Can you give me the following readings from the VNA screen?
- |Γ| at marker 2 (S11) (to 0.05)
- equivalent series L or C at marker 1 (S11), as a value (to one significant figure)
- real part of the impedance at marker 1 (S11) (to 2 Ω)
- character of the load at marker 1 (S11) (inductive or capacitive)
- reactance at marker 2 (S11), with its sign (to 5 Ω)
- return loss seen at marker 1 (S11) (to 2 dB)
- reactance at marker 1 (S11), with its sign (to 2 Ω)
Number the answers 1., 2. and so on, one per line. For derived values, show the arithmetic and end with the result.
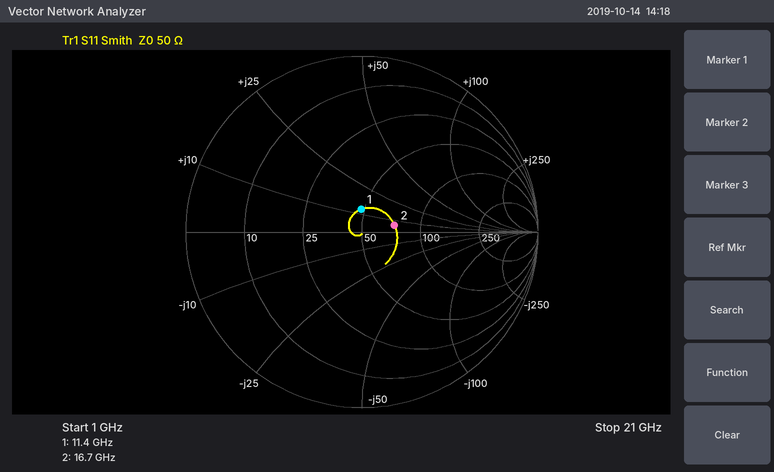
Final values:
1. 0.20
2. L = 12 Ω/(2π × 11.4 GHz) ≈ 168 pH, so 200 pH to one significant figure
3. 48 Ω
4. inductive
5. +5 Ω
6. 18 dB
7. +12 Ω
